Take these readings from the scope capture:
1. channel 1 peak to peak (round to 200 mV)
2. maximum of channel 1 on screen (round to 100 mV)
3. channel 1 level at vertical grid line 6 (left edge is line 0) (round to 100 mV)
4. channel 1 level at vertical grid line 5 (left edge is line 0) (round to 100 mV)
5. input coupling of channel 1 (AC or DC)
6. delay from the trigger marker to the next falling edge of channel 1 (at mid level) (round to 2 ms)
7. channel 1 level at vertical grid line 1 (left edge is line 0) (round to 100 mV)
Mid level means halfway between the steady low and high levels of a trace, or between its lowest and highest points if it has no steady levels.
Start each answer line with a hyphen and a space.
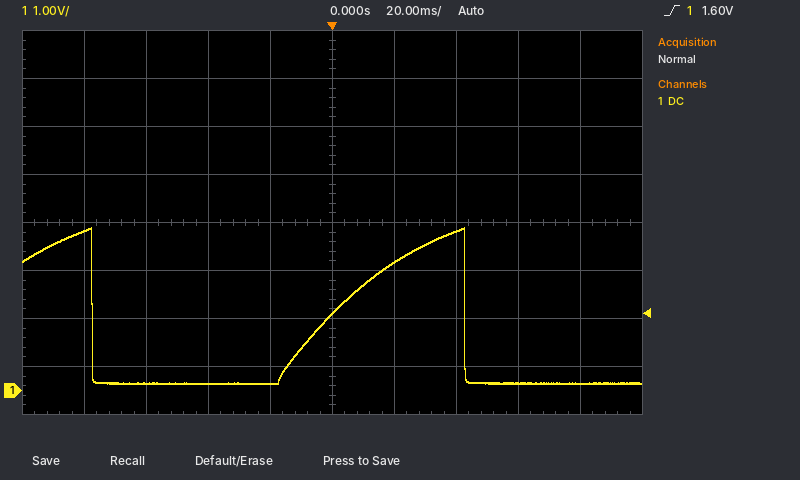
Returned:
- 3.2 V
- 3.4 V
- 2.7 V
- 1.6 V
- DC
- 42 ms
- 3.3 V
